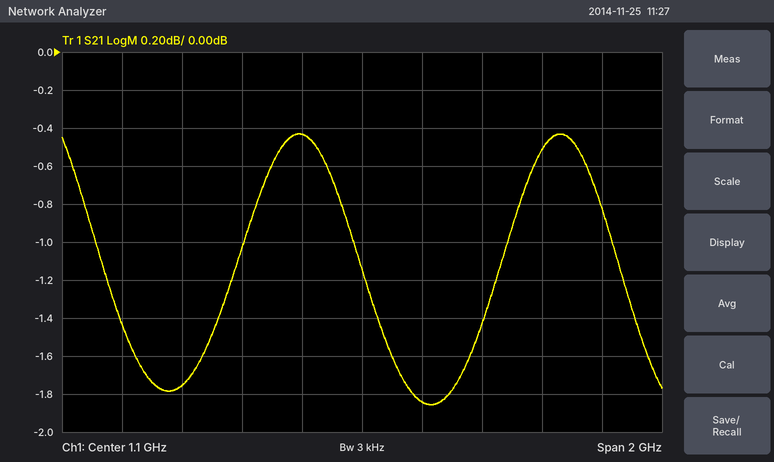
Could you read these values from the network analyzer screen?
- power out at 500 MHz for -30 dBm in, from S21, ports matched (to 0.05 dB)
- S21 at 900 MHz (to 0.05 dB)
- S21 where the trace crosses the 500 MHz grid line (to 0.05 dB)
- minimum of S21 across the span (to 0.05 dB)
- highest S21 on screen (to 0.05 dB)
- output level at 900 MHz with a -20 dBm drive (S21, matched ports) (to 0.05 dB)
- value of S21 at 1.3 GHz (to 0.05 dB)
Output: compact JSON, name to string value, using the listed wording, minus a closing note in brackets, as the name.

{"power out at 500 MHz for -30 dBm in, from S21, ports matched": "-31.75 dBm", "S21 at 900 MHz": "-0.45 dB", "S21 where the trace crosses the 500 MHz grid line": "-1.75 dB", "minimum of S21 across the span": "-1.85 dB", "highest S21 on screen": "-0.45 dB", "output level at 900 MHz with a -20 dBm drive (S21, matched ports)": "-20.45 dBm", "value of S21 at 1.3 GHz": "-1.85 dB"}
